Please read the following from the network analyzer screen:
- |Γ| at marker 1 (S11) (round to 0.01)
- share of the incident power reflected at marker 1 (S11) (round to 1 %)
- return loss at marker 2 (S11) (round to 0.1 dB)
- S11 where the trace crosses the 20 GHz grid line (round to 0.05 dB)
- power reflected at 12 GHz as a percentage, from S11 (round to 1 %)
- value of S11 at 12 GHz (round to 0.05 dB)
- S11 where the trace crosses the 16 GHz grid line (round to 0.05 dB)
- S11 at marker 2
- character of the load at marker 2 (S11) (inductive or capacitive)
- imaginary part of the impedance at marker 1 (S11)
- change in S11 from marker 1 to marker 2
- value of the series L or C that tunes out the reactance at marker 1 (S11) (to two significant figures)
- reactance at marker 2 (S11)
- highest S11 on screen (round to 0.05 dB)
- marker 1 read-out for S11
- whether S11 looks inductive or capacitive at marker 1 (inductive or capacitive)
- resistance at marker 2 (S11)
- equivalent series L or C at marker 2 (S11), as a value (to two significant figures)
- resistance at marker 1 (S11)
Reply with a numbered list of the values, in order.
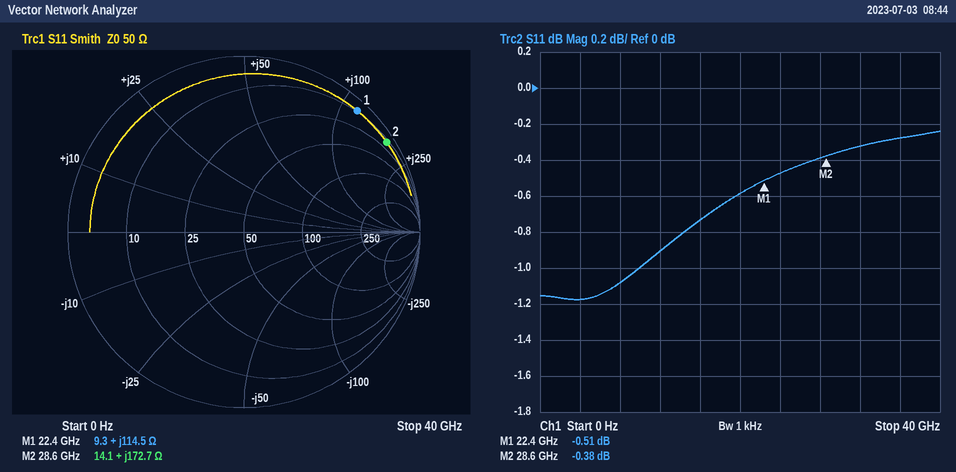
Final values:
1. 0.94
2. 89 %
3. 0.4 dB
4. -0.60 dB
5. 81 %
6. -0.90 dB
7. -0.75 dB
8. -0.38 dB
9. inductive
10. +114.5 Ω
11. 0.13 dB
12. 62 fF
13. +172.7 Ω
14. -0.25 dB
15. -0.51 dB
16. inductive
17. 14.1 Ω
18. 960 pH
19. 9.3 Ω
